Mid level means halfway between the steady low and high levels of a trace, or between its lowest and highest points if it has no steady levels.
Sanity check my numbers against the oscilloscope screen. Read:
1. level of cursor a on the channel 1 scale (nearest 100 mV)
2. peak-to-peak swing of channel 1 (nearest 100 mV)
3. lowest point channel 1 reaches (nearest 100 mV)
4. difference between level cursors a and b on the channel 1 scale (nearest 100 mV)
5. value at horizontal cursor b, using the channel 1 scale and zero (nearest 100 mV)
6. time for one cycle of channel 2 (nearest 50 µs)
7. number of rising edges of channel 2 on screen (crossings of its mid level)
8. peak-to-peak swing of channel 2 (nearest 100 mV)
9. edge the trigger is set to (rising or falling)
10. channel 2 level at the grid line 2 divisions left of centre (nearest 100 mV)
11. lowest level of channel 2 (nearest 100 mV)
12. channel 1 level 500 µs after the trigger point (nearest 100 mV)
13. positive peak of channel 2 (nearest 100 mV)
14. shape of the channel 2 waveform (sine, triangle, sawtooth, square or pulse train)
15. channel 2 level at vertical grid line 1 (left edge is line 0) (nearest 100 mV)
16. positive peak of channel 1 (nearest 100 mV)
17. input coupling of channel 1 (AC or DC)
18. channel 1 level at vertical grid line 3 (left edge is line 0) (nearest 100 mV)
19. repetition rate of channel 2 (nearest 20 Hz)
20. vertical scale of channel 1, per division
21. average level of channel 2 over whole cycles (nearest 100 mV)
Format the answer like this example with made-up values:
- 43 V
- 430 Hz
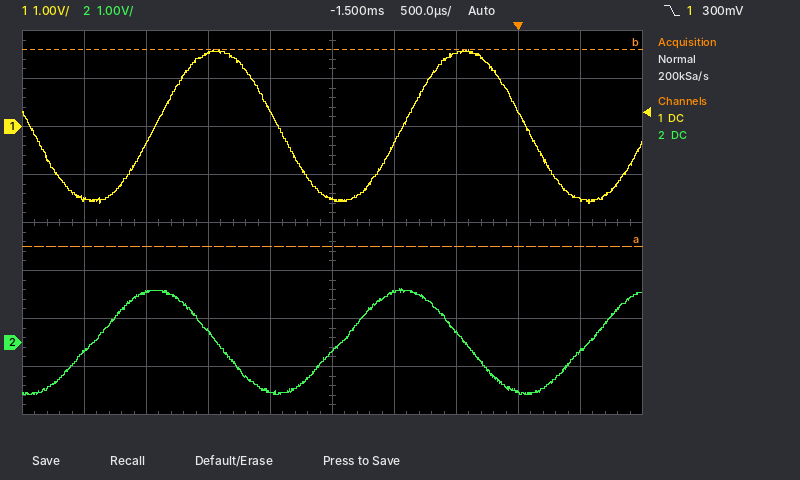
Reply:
- -2.5 V
- 3.2 V
- -1.6 V
- 4.1 V
- 1.6 V
- 2.00 ms
- 3
- 2.2 V
- falling
- 200 mV
- -1.1 V
- -1.5 V
- 1.1 V
- sine
- -200 mV
- 1.6 V
- DC
- 1.5 V
- 500 Hz
- 1 V
- 0.0 V
